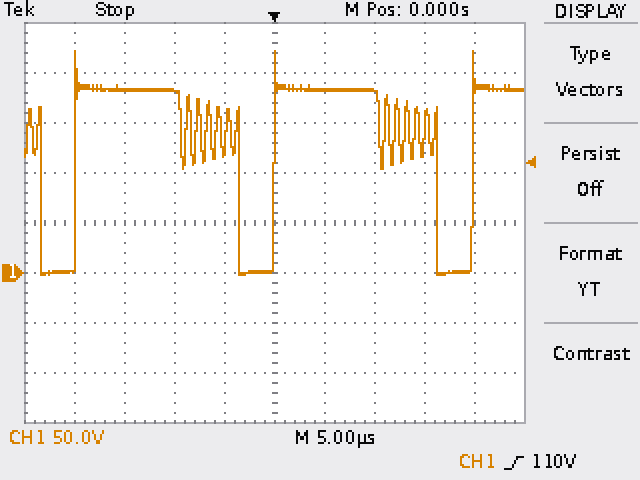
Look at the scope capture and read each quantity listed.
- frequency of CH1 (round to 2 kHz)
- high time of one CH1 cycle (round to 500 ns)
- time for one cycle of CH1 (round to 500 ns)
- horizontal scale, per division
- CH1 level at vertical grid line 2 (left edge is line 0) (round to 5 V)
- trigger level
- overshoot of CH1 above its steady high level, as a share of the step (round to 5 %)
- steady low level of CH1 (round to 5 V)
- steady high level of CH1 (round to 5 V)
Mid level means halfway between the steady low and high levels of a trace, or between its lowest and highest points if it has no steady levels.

50 kHz
16.5 µs
20.0 µs
5 µs
185 V
110 V
20 %
0 V
185 V
